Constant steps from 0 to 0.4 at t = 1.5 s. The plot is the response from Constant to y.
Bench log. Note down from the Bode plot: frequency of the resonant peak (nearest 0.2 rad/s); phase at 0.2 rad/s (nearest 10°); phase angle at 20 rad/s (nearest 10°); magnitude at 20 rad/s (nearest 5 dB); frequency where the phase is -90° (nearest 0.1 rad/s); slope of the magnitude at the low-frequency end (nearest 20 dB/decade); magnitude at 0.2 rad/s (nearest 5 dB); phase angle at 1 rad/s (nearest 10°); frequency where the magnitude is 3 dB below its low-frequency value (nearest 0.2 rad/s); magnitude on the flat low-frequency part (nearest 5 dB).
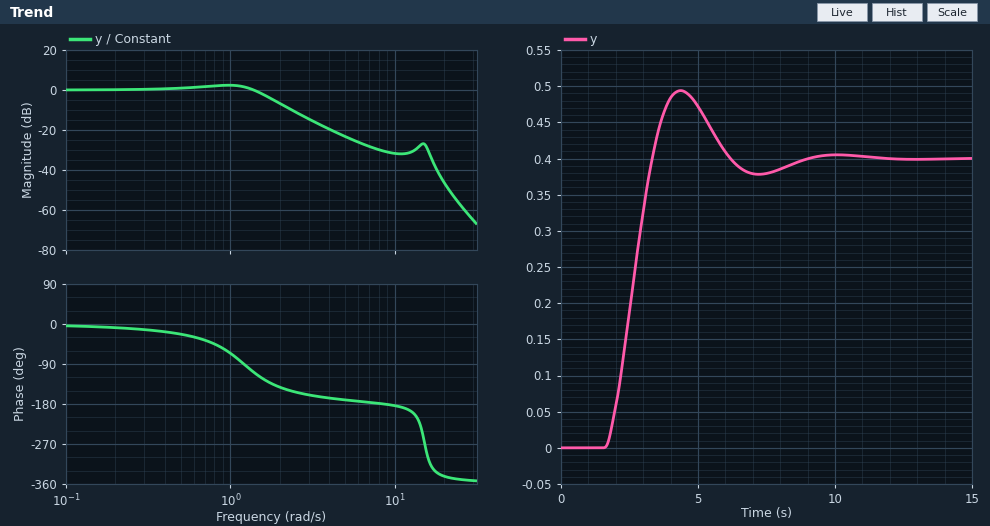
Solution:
1.0 rad/s
-10°
-340°
-45 dB
1.2 rad/s
0 dB/decade
0 dB
-70°
1.6 rad/s
0 dB
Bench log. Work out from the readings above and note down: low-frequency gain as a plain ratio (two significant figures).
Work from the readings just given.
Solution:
1.0
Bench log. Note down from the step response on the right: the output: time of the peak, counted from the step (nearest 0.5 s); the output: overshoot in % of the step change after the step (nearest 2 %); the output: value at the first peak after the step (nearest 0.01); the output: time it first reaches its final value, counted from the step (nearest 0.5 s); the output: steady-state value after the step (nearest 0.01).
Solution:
3.0 s
24 %
0.49
2.0 s
0.40
